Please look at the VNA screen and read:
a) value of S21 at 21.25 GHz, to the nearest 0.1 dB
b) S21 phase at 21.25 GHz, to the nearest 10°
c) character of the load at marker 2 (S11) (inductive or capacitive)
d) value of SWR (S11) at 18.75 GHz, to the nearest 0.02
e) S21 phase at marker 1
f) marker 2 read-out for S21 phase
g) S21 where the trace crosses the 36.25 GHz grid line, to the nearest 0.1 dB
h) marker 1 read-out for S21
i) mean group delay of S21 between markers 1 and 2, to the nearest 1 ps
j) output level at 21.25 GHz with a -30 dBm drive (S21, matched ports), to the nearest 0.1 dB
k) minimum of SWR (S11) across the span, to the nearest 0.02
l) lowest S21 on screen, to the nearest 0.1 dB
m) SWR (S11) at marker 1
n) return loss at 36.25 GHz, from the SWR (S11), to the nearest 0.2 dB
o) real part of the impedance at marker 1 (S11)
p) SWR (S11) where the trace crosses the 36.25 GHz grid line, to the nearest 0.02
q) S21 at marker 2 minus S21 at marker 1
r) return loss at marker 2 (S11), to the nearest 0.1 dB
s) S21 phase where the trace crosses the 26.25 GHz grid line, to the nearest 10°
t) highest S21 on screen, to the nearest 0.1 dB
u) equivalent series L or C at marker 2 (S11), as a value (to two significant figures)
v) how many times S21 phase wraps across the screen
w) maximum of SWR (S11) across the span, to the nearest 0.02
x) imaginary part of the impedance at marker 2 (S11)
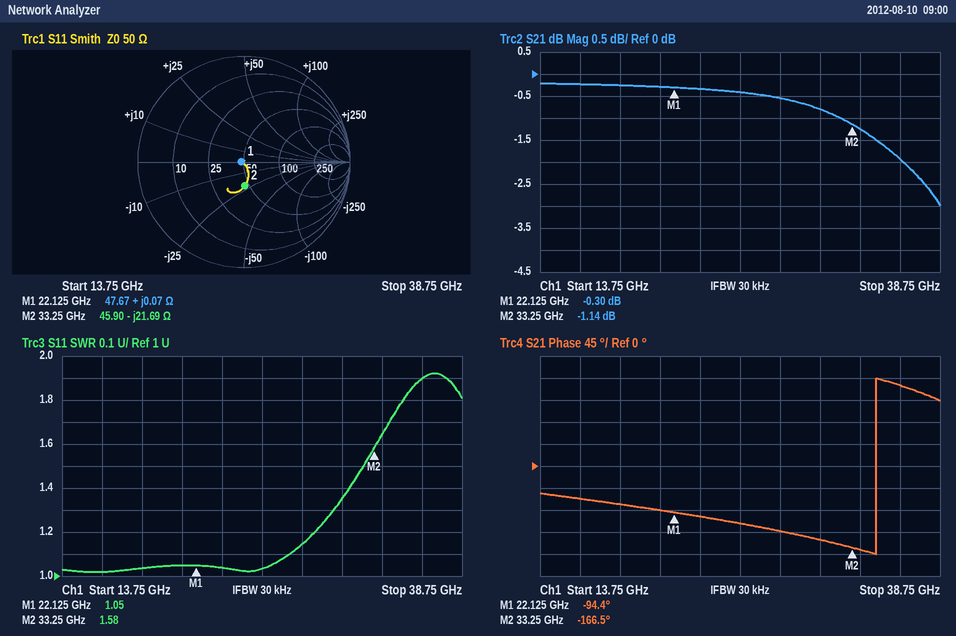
-0.3 dB
-90°
capacitive
1.04
-94.4°
-166.5°
-1.9 dB
-0.30 dB
18 ps
-30.3 dBm
1.02
-3.0 dB
1.05
10.2 dB
47.67 Ω
1.90
-0.84 dB
13.0 dB
-120°
-0.2 dB
220 fF
1
1.92
-21.69 Ω
